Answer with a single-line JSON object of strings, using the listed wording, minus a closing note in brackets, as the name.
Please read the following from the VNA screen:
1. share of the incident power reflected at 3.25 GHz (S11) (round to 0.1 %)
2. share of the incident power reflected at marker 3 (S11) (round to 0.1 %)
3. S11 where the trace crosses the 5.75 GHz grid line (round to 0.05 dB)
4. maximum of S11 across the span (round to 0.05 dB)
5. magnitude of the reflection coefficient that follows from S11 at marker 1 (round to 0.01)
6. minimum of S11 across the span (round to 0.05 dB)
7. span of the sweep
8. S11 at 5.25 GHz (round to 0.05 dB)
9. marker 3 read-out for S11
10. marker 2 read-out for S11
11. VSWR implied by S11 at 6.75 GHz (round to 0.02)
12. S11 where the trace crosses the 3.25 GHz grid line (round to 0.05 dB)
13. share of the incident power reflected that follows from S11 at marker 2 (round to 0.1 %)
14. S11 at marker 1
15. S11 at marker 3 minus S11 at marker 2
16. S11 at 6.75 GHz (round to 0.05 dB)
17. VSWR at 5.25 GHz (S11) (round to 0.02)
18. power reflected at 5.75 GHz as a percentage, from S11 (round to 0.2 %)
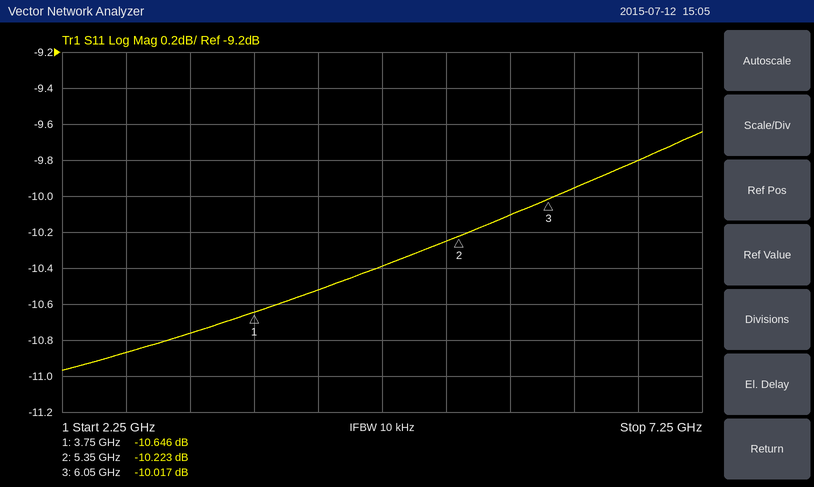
{"share of the incident power reflected at 3.25 GHz (S11)": "8.4 %", "share of the incident power reflected at marker 3 (S11)": "10.0 %", "S11 where the trace crosses the 5.75 GHz grid line": "-10.10 dB", "maximum of S11 across the span": "-9.65 dB", "magnitude of the reflection coefficient that follows from S11 at marker 1": "0.29", "minimum of S11 across the span": "-10.95 dB", "span of the sweep": "5 GHz", "S11 at 5.25 GHz": "-10.25 dB", "marker 3 read-out for S11": "-10.017 dB", "marker 2 read-out for S11": "-10.223 dB", "VSWR implied by S11 at 6.75 GHz": "1.96", "S11 where the trace crosses the 3.25 GHz grid line": "-10.75 dB", "share of the incident power reflected that follows from S11 at marker 2": "9.5 %", "S11 at marker 1": "-10.646 dB", "S11 at marker 3 minus S11 at marker 2": "0.206 dB", "S11 at 6.75 GHz": "-9.80 dB", "VSWR at 5.25 GHz (S11)": "1.88", "power reflected at 5.75 GHz as a percentage, from S11": "9.8 %"}
